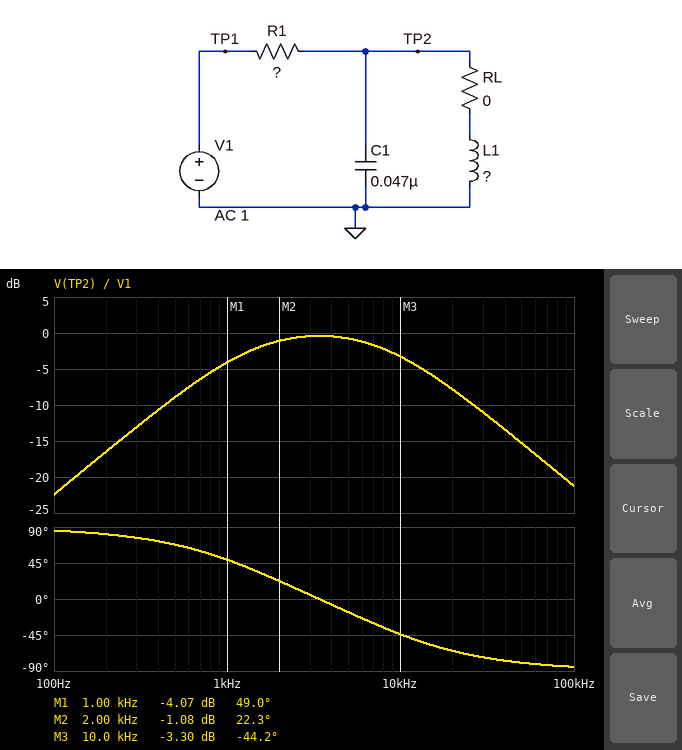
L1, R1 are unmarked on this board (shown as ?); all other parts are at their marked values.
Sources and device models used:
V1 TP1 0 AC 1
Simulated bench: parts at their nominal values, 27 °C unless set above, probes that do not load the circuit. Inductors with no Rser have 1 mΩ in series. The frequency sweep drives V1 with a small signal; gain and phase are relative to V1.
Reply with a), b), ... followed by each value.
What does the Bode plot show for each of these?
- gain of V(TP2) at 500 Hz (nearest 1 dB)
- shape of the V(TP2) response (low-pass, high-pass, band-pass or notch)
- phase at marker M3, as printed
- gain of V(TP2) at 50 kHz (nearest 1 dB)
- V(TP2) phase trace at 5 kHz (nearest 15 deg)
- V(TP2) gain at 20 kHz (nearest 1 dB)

a) -9 dB
b) band-pass
c) -44.2 deg
d) -15 dB
e) -15 deg
f) -8 dB
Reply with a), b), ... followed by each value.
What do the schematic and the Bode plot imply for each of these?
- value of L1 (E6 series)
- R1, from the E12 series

a) 47 mH
b) 390 Ω
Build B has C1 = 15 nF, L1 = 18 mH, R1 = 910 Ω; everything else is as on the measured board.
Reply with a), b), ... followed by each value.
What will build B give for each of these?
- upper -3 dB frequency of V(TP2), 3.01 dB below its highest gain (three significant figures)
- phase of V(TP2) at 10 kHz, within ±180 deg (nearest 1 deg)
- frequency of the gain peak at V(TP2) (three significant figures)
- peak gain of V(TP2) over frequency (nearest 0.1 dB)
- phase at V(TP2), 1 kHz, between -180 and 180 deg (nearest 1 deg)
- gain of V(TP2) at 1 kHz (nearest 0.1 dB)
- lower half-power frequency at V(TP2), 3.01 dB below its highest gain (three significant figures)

a) 16.2 kHz
b) -3 deg
c) 9.69 kHz
d) 1.0 dB
e) 84 deg
f) -18.1 dB
g) 5.80 kHz
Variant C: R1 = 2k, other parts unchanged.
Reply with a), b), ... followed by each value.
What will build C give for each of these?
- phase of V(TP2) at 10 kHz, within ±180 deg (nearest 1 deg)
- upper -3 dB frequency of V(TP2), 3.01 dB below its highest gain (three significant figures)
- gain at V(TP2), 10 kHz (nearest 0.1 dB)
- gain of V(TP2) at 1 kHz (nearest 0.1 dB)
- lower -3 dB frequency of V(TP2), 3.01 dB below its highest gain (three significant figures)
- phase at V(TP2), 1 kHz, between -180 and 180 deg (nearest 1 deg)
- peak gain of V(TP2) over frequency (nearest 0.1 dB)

a) -79 deg
b) 4.31 kHz
c) -14.5 dB
d) -15.9 dB
e) 2.66 kHz
f) 81 deg
g) 0.2 dB
